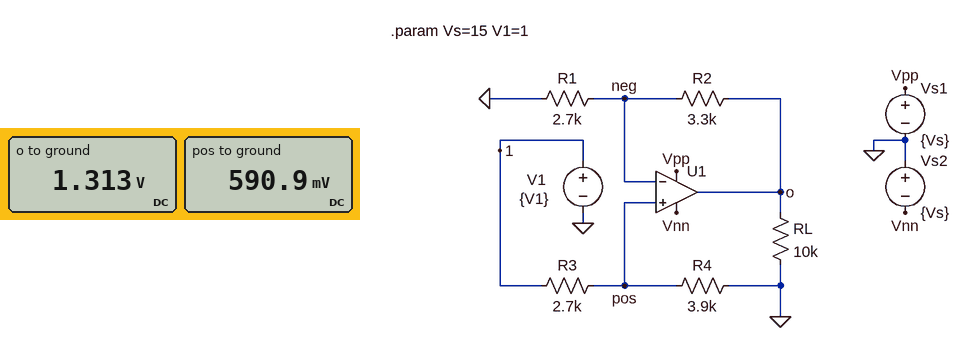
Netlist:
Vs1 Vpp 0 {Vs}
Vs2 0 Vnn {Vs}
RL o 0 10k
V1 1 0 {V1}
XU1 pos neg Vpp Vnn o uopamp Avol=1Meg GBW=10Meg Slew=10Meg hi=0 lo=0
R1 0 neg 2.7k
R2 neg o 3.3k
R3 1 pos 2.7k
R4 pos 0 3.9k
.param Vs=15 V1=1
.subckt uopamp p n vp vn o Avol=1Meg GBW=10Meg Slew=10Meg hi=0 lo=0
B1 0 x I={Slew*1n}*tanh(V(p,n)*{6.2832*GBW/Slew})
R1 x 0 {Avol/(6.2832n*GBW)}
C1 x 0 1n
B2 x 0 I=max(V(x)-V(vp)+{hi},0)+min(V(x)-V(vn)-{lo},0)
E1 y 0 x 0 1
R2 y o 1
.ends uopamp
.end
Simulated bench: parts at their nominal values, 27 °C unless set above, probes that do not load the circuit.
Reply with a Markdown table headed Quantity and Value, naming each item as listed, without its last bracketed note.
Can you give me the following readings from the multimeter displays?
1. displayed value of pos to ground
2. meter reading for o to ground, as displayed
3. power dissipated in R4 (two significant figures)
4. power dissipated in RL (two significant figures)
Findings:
| Quantity | Value |
|---|---|
| displayed value of pos to ground | 590.9 mV |
| meter reading for o to ground, as displayed | 1.313 V |
| power dissipated in R4 | 90 µW |
| power dissipated in RL | 170 µW |
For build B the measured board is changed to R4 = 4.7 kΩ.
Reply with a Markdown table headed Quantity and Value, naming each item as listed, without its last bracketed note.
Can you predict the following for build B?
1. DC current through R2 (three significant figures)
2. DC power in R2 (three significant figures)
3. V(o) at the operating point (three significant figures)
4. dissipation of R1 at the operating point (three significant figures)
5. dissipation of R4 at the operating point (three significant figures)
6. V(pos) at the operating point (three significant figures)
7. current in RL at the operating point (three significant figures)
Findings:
| Quantity | Value |
|---|---|
| DC current through R2 | 235 µA |
| DC power in R2 | 183 µW |
| V(o) at the operating point | 1.41 V |
| dissipation of R1 at the operating point | 149 µW |
| dissipation of R4 at the operating point | 85.8 µW |
| V(pos) at the operating point | 635 mV |
| current in RL at the operating point | 141 µA |
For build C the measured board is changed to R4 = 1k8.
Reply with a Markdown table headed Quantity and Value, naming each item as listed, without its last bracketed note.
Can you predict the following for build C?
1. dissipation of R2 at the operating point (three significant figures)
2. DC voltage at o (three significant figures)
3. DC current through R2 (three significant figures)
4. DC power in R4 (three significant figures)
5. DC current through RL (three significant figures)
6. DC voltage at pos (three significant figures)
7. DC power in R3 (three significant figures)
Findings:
| Quantity | Value |
|---|---|
| dissipation of R2 at the operating point | 72.4 µW |
| DC voltage at o | 889 mV |
| DC current through R2 | 148 µA |
| DC power in R4 | 88.9 µW |
| DC current through RL | 88.9 µA |
| DC voltage at pos | 400 mV |
| DC power in R3 | 133 µW |
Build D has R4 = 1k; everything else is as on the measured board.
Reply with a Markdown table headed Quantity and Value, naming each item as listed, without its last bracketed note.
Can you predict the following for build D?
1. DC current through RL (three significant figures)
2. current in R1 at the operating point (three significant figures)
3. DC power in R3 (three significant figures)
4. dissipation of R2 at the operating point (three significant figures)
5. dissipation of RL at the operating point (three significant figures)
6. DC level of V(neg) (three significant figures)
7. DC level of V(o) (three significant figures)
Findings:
| Quantity | Value |
|---|---|
| DC current through RL | 60.1 µA |
| current in R1 at the operating point | 100 µA |
| DC power in R3 | 197 µW |
| dissipation of R2 at the operating point | 33.1 µW |
| dissipation of RL at the operating point | 36.1 µW |
| DC level of V(neg) | 270 mV |
| DC level of V(o) | 601 mV |
